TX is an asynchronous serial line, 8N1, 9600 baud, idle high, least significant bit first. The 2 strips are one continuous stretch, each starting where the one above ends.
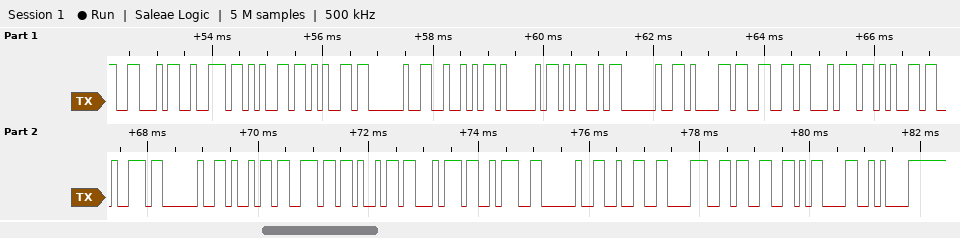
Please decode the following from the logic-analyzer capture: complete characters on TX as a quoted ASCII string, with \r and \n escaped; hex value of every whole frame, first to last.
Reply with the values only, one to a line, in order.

"Free RAM after init: 283\r\n"
46 72 65 65 20 52 41 4D 20 61 66 74 65 72 20 69 6E 69 74 3A 20 32 38 33 0D 0A
